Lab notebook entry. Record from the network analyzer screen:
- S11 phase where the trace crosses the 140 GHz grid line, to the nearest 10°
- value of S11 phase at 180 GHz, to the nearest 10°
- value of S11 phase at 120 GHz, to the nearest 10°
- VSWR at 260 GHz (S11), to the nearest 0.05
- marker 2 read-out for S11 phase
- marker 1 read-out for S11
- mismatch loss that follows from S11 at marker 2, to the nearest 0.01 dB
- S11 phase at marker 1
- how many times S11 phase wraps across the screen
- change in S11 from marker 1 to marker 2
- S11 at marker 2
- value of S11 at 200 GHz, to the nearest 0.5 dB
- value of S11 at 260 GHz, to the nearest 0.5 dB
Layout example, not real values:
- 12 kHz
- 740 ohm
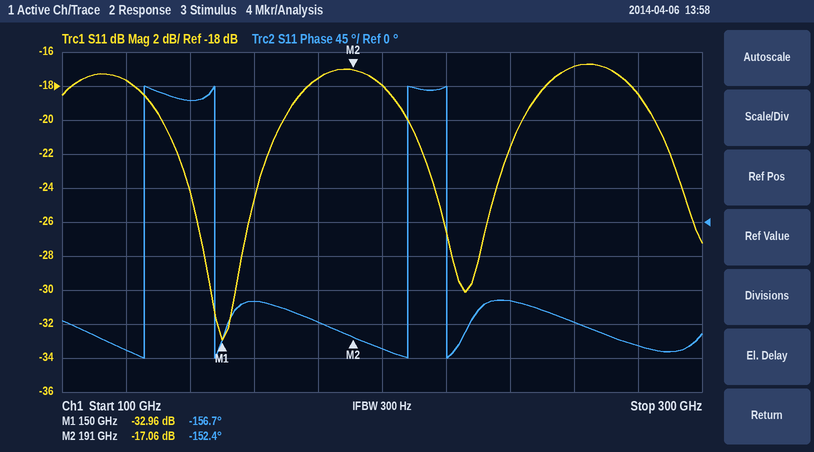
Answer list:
- 160°
- -130°
- -170°
- 1.35
- -152.4°
- -32.96 dB
- 0.09 dB
- -156.7°
- 4
- 15.90 dB
- -17.06 dB
- -18.0 dB
- -17.0 dB
